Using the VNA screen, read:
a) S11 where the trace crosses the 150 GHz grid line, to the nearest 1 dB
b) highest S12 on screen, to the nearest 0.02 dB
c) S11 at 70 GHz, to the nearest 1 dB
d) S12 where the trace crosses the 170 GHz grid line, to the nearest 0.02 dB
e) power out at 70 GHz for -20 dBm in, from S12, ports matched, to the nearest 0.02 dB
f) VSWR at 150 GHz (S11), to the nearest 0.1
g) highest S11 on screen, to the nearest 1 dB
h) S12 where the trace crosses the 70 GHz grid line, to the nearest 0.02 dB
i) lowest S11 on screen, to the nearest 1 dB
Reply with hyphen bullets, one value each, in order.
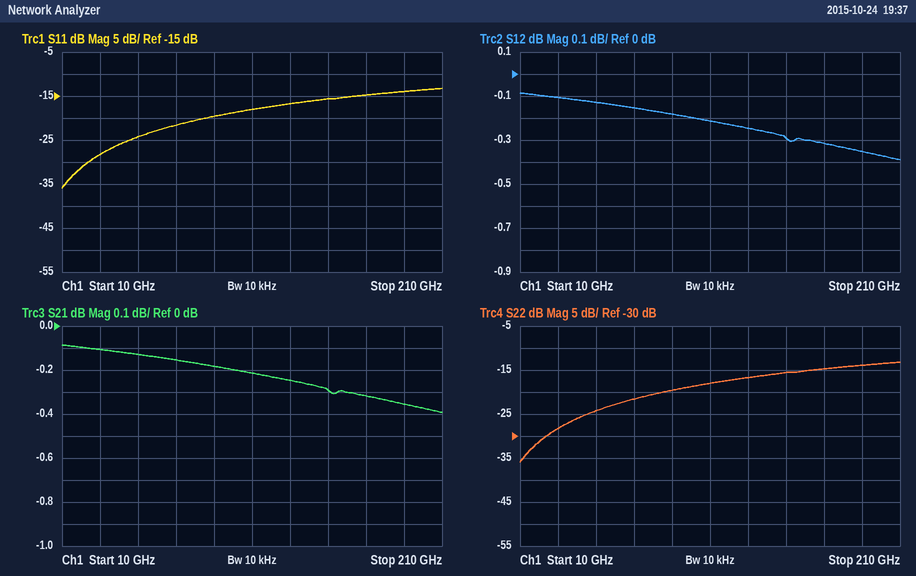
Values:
- -16 dB
- -0.08 dB
- -22 dB
- -0.32 dB
- -20.16 dBm
- 1.4
- -13 dB
- -0.16 dB
- -36 dB
